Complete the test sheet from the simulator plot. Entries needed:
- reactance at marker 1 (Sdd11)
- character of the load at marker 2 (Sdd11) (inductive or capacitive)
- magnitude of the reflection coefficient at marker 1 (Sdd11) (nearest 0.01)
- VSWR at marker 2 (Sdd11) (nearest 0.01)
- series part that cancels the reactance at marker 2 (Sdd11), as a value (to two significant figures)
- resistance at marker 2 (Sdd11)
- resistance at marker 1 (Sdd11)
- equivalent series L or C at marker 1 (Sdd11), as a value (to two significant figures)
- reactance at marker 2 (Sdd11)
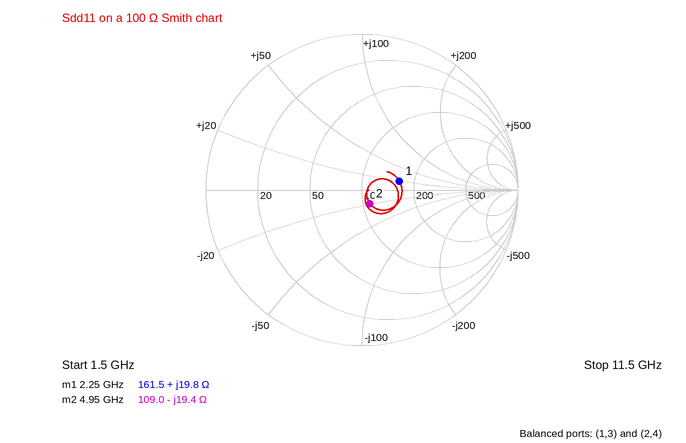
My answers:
+19.8 Ω
capacitive
0.25
1.23
620 pH
109.0 Ω
161.5 Ω
1.4 nH
-19.4 Ω
